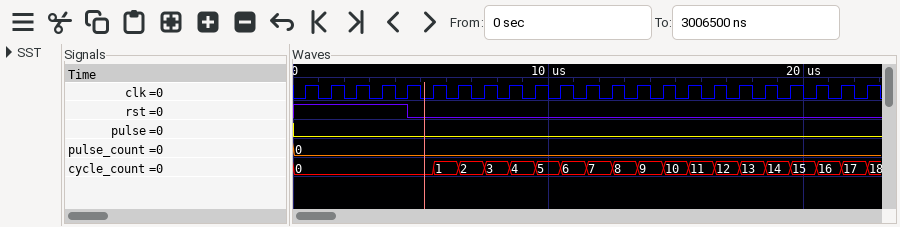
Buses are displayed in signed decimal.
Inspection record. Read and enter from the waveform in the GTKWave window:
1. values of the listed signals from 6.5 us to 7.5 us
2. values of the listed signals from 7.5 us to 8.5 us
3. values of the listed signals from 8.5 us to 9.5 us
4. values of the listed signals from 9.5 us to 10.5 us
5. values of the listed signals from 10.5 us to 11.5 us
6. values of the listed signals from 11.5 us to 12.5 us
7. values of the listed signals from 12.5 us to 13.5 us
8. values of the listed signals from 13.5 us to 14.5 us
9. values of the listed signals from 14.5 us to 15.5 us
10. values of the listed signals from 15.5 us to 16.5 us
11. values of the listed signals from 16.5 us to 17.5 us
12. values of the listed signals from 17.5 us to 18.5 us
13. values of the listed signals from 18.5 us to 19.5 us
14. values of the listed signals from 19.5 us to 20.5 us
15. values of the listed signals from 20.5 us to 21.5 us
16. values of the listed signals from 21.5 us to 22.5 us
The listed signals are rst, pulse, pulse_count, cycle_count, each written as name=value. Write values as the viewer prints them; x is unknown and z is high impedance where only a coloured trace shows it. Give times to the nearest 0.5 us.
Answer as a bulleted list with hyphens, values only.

- rst=0, pulse=0, pulse_count=0, cycle_count=2
- rst=0, pulse=0, pulse_count=0, cycle_count=3
- rst=0, pulse=0, pulse_count=0, cycle_count=4
- rst=0, pulse=0, pulse_count=0, cycle_count=5
- rst=0, pulse=0, pulse_count=0, cycle_count=6
- rst=0, pulse=0, pulse_count=0, cycle_count=7
- rst=0, pulse=0, pulse_count=0, cycle_count=8
- rst=0, pulse=0, pulse_count=0, cycle_count=9
- rst=0, pulse=0, pulse_count=0, cycle_count=10
- rst=0, pulse=0, pulse_count=0, cycle_count=11
- rst=0, pulse=0, pulse_count=0, cycle_count=12
- rst=0, pulse=0, pulse_count=0, cycle_count=13
- rst=0, pulse=0, pulse_count=0, cycle_count=14
- rst=0, pulse=0, pulse_count=0, cycle_count=15
- rst=0, pulse=0, pulse_count=0, cycle_count=16
- rst=0, pulse=0, pulse_count=0, cycle_count=17
